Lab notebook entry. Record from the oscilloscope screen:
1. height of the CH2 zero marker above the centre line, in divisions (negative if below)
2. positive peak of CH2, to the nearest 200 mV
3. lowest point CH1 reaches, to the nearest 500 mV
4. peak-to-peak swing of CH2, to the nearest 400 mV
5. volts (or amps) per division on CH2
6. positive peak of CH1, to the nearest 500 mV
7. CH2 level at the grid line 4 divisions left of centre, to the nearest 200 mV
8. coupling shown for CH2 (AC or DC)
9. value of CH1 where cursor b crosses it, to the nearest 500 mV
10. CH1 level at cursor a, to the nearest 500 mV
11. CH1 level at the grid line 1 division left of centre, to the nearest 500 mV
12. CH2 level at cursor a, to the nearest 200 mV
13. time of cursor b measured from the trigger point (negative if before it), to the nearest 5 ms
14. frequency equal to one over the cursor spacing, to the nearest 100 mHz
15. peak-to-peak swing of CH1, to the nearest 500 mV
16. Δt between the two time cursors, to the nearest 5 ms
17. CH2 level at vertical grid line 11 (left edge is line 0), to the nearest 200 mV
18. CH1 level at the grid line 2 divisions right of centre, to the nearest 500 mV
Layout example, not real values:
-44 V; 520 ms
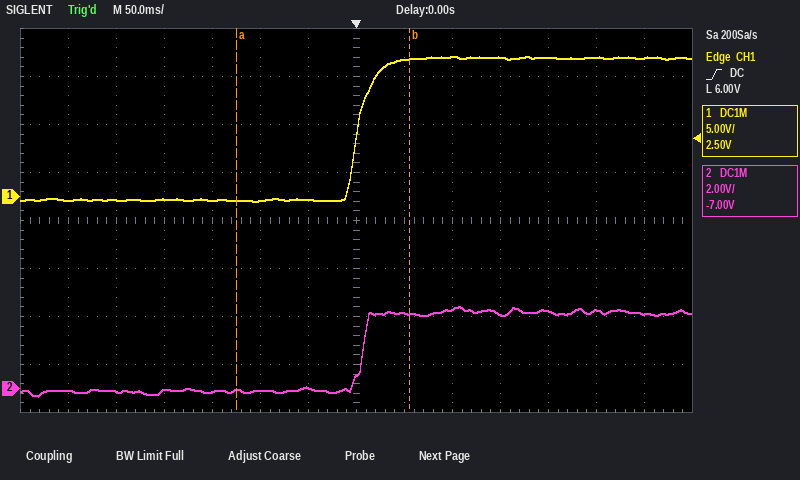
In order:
-3.5 div; 3.4 V; -500 mV; 3.6 V; 2 V; 14.5 V; 0.0 V; DC; 14.5 V; -500 mV; -500 mV; 0.0 V; +55 ms; 5.6 Hz; 15.0 V; 180 ms; 3.2 V; 14.5 V
